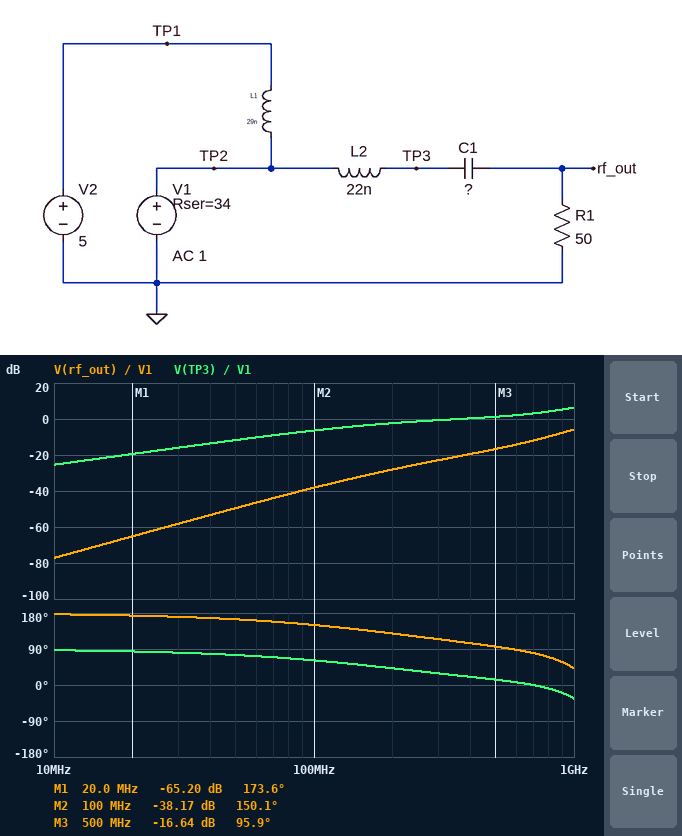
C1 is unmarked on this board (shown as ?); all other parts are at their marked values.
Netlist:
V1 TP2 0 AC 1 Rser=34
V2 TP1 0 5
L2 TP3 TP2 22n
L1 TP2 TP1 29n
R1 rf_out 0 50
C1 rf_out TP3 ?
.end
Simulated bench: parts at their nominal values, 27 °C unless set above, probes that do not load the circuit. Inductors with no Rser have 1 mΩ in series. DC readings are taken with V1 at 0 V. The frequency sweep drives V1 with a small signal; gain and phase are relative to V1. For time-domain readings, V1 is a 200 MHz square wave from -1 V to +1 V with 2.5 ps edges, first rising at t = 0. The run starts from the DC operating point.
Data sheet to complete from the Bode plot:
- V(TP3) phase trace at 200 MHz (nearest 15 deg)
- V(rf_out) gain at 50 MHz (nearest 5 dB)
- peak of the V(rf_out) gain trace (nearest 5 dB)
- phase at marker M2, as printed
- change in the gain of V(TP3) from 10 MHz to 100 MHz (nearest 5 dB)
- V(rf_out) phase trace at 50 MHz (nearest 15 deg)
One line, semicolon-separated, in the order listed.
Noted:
45 deg; -50 dB; -5 dB; 150.1 deg; 20 dB; 165 deg
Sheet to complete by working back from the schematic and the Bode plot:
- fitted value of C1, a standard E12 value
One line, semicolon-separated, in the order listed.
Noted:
820 fF
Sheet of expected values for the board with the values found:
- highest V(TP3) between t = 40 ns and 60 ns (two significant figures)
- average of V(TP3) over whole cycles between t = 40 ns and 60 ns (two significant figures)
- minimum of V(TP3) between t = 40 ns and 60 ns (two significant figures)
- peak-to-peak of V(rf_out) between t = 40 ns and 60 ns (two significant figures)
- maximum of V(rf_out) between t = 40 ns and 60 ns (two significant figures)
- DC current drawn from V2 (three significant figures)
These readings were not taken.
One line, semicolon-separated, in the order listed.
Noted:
7.3 V; 5.0 V; 2.7 V; 770 mV; 390 mV; 147 mA
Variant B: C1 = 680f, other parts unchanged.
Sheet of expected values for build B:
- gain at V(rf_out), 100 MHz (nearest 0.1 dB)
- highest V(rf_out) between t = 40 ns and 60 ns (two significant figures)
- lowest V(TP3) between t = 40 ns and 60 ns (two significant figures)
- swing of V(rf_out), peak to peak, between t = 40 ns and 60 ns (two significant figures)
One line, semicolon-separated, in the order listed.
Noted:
-39.8 dB; 360 mV; 2.6 V; 720 mV
